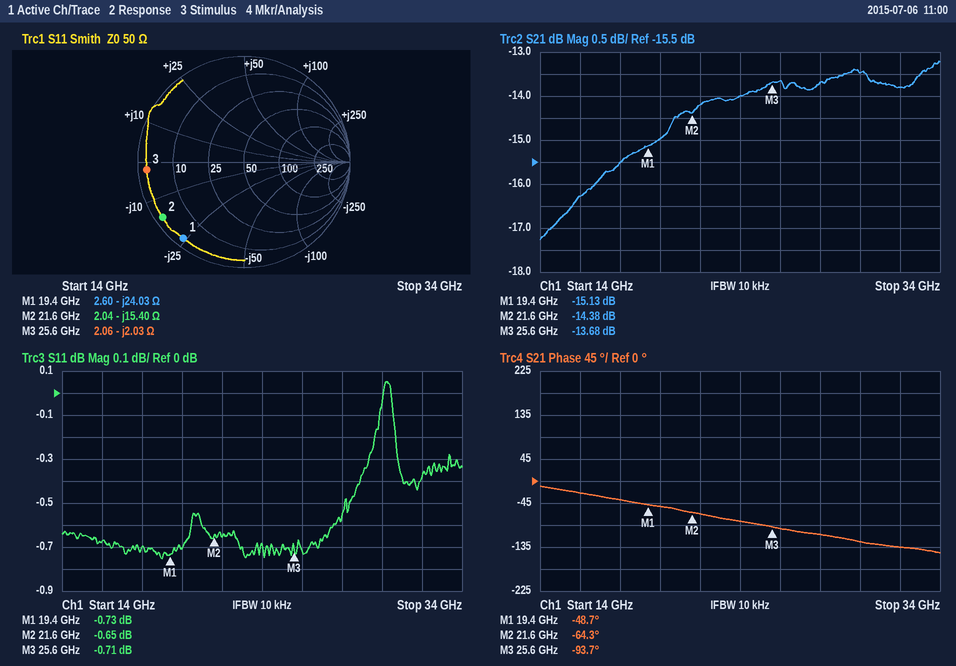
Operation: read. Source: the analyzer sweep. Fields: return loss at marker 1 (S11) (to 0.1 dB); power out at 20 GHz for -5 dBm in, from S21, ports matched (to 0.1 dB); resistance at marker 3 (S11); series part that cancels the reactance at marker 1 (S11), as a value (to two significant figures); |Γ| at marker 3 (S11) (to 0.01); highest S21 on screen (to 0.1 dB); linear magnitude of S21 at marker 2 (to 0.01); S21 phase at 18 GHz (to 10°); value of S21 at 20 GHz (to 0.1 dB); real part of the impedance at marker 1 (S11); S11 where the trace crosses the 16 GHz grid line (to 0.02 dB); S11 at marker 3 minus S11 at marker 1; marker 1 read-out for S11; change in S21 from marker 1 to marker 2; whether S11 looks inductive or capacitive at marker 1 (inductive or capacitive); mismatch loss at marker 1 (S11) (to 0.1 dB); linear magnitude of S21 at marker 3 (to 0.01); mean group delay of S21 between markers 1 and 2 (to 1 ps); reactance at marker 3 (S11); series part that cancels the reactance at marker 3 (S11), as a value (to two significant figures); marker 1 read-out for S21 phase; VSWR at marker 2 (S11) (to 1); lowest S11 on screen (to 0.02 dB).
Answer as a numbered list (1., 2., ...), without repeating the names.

1. 0.7 dB
2. -20.0 dBm
3. 2.06 Ω
4. 200 pH
5. 0.92
6. -13.2 dB
7. 0.19
8. -40°
9. -15.0 dB
10. 2.60 Ω
11. -0.68 dB
12. 0.02 dB
13. -0.73 dB
14. 0.75 dB
15. capacitive
16. 8.1 dB
17. 0.21
18. 20 ps
19. -2.03 Ω
20. 13 pH
21. -48.7°
22. 27
23. -0.76 dB
